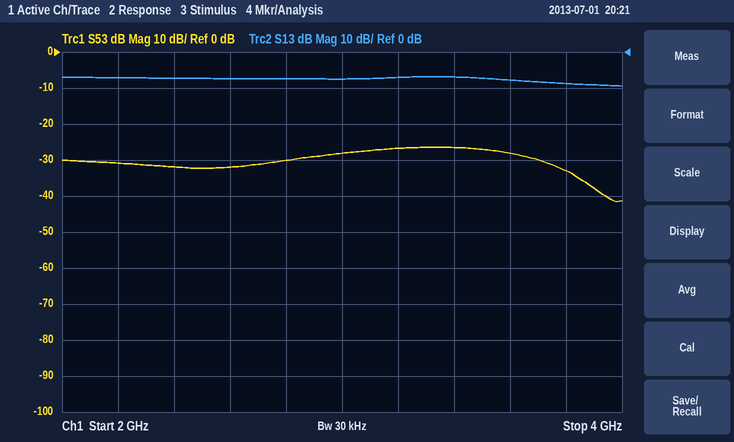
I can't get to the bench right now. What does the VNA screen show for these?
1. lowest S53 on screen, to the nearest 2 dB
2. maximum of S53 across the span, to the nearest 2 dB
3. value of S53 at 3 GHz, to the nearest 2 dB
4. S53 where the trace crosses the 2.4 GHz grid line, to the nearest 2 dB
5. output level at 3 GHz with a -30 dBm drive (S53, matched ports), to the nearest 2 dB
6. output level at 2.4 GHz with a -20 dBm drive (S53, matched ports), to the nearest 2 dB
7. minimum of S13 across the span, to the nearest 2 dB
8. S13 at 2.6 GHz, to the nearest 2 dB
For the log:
-42 dB
-26 dB
-28 dB
-32 dB
-58 dBm
-52 dBm
-10 dB
-8 dB
